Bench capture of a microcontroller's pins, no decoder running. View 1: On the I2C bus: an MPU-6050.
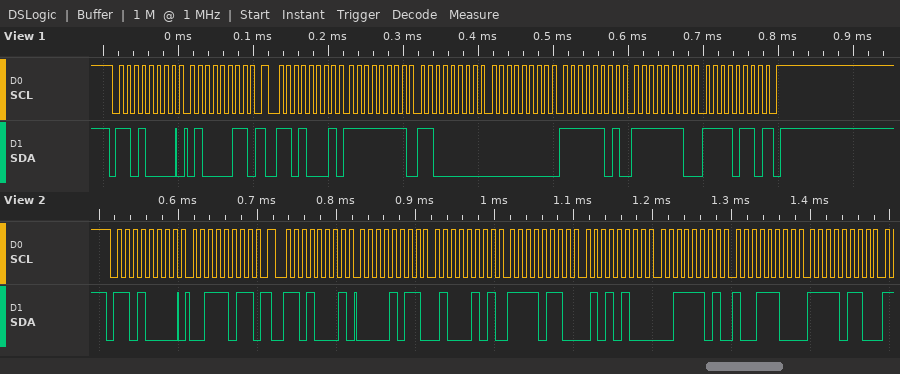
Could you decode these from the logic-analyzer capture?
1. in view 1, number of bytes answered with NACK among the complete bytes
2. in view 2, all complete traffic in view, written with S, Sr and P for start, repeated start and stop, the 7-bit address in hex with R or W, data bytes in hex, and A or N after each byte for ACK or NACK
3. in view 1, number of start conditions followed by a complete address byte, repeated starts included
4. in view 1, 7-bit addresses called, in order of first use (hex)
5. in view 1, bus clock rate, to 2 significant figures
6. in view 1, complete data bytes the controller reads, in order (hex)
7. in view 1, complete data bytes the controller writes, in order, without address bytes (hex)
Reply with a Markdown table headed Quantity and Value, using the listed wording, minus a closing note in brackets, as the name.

| Quantity | Value |
|---|---|
| in view 1, number of bytes answered with NACK among the complete bytes | 1 |
| in view 2, all complete traffic in view, written with S, Sr and P for start, repeated start and stop, the 7-bit address in hex with R or W, data bytes in hex, and A or N after each byte for ACK or NACK | S 68W A 3B A Sr 68R A 0B A 45 A F6 A 54 A 3D A 9C A F6 A |
| in view 1, number of start conditions followed by a complete address byte, repeated starts included | 2 |
| in view 1, 7-bit addresses called, in order of first use | 0x68 |
| in view 1, bus clock rate, to 2 significant figures | 100 kHz |
| in view 1, complete data bytes the controller reads, in order | FF C0 00 FD FE F6 |
| in view 1, complete data bytes the controller writes, in order, without address bytes | 43 |
